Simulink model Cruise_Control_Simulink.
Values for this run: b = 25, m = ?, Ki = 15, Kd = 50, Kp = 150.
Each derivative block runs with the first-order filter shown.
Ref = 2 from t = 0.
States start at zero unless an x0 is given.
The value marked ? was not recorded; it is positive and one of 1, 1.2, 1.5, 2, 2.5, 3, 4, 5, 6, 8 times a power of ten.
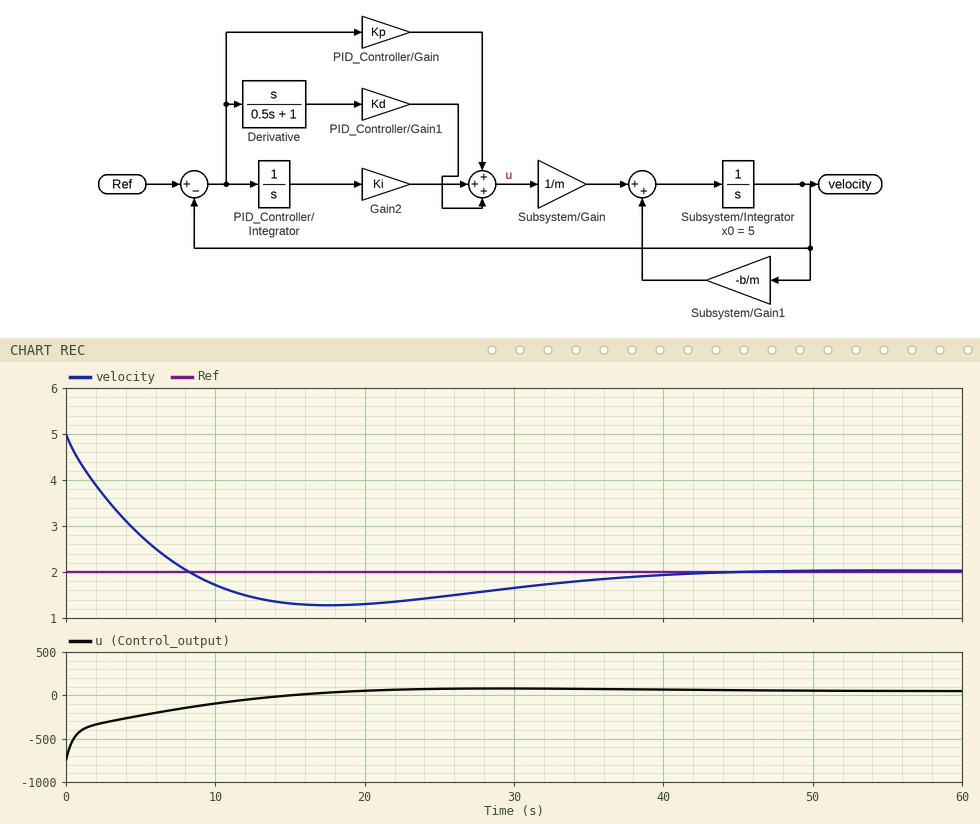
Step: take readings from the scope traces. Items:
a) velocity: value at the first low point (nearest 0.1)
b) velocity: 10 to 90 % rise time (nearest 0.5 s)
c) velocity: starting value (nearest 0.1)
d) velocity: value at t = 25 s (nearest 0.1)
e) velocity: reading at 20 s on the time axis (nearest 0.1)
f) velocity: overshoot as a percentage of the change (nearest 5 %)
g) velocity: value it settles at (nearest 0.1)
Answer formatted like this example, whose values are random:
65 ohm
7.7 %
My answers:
1.3
6.5 s
5.0
1.5
1.3
25 %
2.0
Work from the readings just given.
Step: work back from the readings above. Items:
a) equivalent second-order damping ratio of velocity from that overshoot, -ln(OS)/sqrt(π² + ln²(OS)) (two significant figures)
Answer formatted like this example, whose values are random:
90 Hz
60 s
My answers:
0.40
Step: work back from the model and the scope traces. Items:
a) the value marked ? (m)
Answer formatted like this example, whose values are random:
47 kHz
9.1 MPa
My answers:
1000
